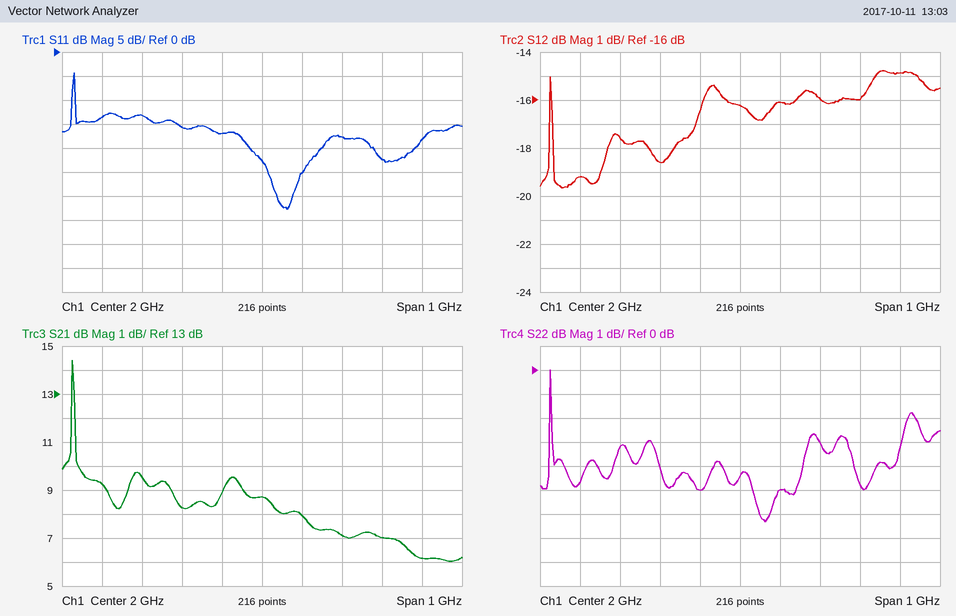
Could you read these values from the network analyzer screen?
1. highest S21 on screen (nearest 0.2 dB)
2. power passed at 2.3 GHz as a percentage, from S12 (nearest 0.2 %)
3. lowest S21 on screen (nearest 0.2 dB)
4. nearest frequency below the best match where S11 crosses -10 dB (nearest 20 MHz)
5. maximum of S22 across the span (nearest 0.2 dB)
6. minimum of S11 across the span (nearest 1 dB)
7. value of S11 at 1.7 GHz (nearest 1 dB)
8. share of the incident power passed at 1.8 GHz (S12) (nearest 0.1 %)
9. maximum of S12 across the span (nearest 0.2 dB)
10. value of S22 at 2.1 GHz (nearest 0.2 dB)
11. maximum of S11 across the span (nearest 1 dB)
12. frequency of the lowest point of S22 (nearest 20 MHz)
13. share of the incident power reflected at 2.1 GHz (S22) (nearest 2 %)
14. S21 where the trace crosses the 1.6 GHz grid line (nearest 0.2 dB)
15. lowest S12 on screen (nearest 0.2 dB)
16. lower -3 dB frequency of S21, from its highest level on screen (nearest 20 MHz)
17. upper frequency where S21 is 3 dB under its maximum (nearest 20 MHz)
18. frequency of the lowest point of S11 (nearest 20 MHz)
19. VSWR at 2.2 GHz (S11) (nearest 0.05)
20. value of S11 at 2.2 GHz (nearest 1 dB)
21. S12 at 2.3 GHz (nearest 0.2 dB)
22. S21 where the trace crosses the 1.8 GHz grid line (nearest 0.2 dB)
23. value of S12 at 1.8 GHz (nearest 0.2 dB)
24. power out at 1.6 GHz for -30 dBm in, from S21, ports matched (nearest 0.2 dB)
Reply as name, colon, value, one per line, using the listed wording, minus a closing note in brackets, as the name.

highest S21 on screen: 14.4 dB
power passed at 2.3 GHz as a percentage, from S12: 2.6 %
lowest S21 on screen: 6.0 dB
nearest frequency below the best match where S11 crosses -10 dB: 1.54 GHz
maximum of S22 across the span: 0.0 dB
minimum of S11 across the span: -33 dB
value of S11 at 1.7 GHz: -13 dB
share of the incident power passed at 1.8 GHz (S12): 1.4 %
maximum of S12 across the span: -14.8 dB
value of S22 at 2.1 GHz: -5.0 dB
maximum of S11 across the span: -4 dB
frequency of the lowest point of S22: 2.06 GHz
share of the incident power reflected at 2.1 GHz (S22): 32 %
S21 where the trace crosses the 1.6 GHz grid line: 9.2 dB
lowest S12 on screen: -19.6 dB
lower -3 dB frequency of S21, from its highest level on screen: 1.52 GHz
upper frequency where S21 is 3 dB under its maximum: 1.54 GHz
frequency of the lowest point of S11: 2.06 GHz
VSWR at 2.2 GHz (S11): 1.30
value of S11 at 2.2 GHz: -18 dB
S12 at 2.3 GHz: -16.0 dB
S21 where the trace crosses the 1.8 GHz grid line: 8.2 dB
value of S12 at 1.8 GHz: -18.6 dB
power out at 1.6 GHz for -30 dBm in, from S21, ports matched: -20.8 dBm
